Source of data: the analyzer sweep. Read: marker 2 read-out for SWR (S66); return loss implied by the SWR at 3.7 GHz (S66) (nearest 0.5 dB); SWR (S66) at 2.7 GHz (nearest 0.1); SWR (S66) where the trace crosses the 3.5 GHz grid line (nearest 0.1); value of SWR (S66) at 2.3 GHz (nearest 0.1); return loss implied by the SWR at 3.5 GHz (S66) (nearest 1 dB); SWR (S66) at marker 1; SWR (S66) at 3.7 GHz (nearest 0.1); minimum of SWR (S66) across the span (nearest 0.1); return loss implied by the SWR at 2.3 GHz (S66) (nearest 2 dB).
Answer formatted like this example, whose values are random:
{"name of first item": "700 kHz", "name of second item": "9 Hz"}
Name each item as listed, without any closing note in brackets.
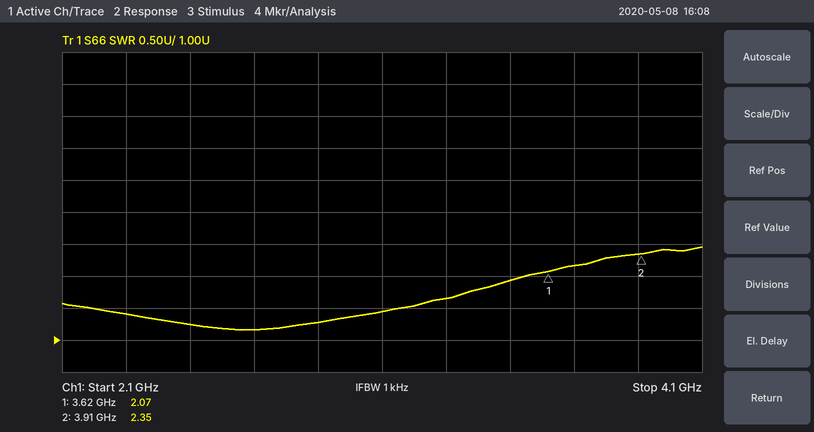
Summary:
{"marker 2 read-out for SWR": "2.35", "return loss implied by the SWR at 3.7 GHz (S66)": "8.5 dB", "SWR (S66) at 2.7 GHz": "1.2", "SWR (S66) where the trace crosses the 3.5 GHz grid line": "1.9", "value of SWR (S66) at 2.3 GHz": "1.4", "return loss implied by the SWR at 3.5 GHz (S66)": "10 dB", "SWR (S66) at marker 1": "2.07", "SWR (S66) at 3.7 GHz": "2.2", "minimum of SWR (S66) across the span": "1.2", "return loss implied by the SWR at 2.3 GHz (S66)": "16 dB"}
